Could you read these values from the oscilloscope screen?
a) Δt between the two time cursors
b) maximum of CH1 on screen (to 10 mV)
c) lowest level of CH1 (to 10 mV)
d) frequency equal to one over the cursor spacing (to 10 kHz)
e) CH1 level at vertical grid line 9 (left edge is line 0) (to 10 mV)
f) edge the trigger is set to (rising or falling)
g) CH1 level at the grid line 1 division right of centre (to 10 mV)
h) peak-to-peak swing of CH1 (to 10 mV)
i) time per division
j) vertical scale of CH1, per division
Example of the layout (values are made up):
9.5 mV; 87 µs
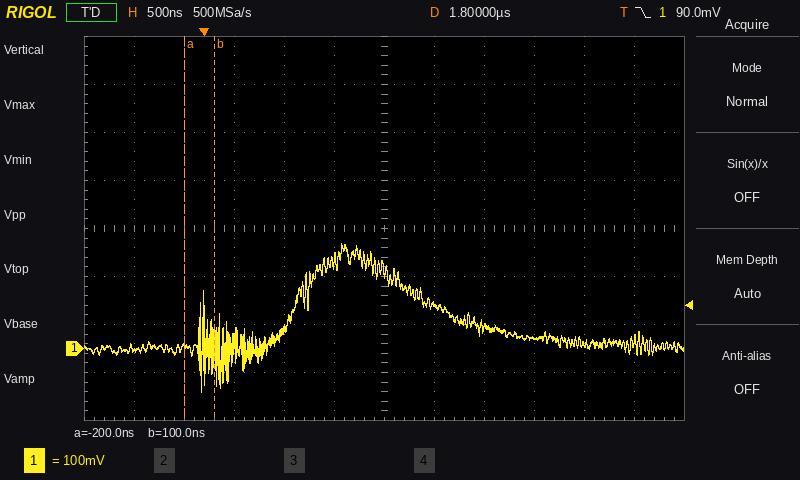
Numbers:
300 ns; 220 mV; -90 mV; 3.33 MHz; 20 mV; falling; 90 mV; 310 mV; 500 ns; 100 mV
